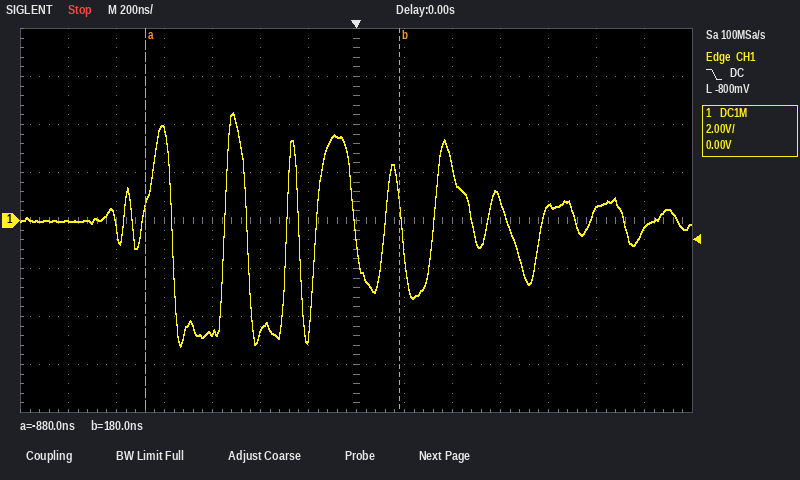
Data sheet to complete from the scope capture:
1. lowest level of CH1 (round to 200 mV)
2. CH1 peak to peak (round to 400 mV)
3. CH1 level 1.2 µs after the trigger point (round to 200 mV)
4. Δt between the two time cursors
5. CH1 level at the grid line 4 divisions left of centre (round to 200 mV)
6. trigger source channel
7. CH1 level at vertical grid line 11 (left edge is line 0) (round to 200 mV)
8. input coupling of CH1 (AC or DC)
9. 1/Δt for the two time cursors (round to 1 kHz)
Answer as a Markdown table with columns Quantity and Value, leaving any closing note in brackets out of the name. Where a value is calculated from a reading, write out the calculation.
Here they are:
| Quantity | Value |
|---|---|
| lowest level of CH1 | -5.2 V |
| CH1 peak to peak | 9.6 V |
| CH1 level 1.2 µs after the trigger point | -400 mV |
| Δt between the two time cursors | 180 ns − (-880 ns) = 1.06 µs |
| CH1 level at the grid line 4 divisions left of centre | 3.8 V |
| trigger source channel | CH1 |
| CH1 level at vertical grid line 11 (left edge is line 0) | 600 mV |
| input coupling of CH1 | DC |
| 1/Δt for the two time cursors | 1 / 1.06 µs ≈ 943 kHz |
